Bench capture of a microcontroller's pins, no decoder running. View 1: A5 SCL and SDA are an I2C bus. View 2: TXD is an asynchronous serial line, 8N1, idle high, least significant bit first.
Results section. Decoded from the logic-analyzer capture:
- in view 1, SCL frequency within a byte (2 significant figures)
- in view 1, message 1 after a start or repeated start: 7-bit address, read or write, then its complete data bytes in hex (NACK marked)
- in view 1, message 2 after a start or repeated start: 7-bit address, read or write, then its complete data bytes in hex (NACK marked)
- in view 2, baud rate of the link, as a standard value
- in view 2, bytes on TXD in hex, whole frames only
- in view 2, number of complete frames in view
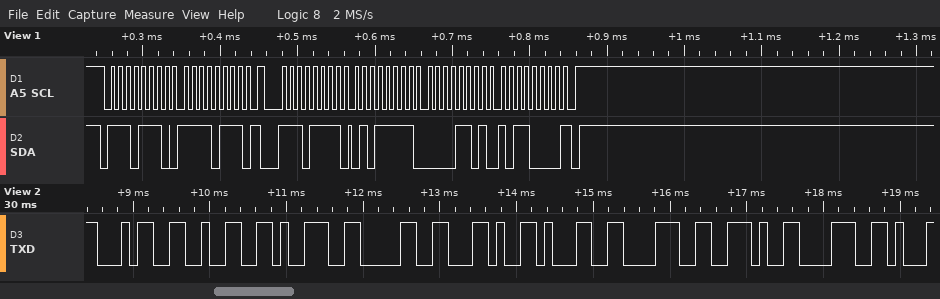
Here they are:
100 kHz
0x77 write: F7
0x77 read: 5F 0D B0 NACK
9600 baud
34 32 39 30 2C 31 38 2E 38
9
